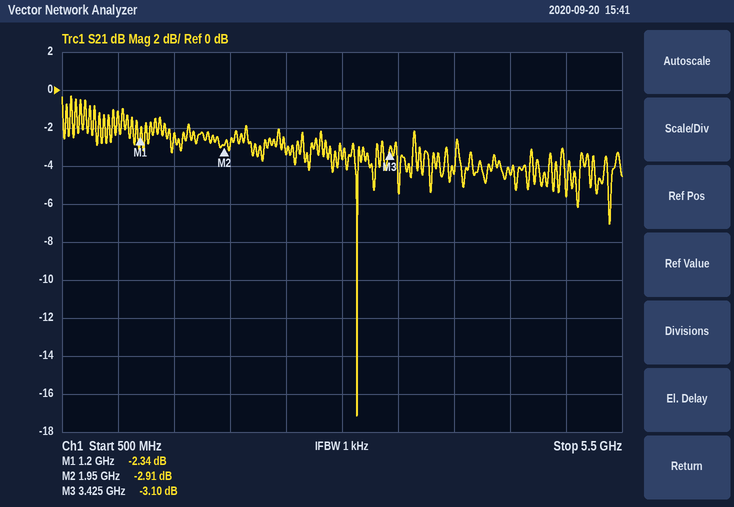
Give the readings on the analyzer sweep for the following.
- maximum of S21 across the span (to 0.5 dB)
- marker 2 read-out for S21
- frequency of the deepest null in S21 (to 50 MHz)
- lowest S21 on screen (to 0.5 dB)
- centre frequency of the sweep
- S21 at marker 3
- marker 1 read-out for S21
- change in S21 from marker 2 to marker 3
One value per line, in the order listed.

-0.5 dB
-2.91 dB
3.15 GHz
-17.0 dB
3 GHz
-3.10 dB
-2.34 dB
-0.19 dB
